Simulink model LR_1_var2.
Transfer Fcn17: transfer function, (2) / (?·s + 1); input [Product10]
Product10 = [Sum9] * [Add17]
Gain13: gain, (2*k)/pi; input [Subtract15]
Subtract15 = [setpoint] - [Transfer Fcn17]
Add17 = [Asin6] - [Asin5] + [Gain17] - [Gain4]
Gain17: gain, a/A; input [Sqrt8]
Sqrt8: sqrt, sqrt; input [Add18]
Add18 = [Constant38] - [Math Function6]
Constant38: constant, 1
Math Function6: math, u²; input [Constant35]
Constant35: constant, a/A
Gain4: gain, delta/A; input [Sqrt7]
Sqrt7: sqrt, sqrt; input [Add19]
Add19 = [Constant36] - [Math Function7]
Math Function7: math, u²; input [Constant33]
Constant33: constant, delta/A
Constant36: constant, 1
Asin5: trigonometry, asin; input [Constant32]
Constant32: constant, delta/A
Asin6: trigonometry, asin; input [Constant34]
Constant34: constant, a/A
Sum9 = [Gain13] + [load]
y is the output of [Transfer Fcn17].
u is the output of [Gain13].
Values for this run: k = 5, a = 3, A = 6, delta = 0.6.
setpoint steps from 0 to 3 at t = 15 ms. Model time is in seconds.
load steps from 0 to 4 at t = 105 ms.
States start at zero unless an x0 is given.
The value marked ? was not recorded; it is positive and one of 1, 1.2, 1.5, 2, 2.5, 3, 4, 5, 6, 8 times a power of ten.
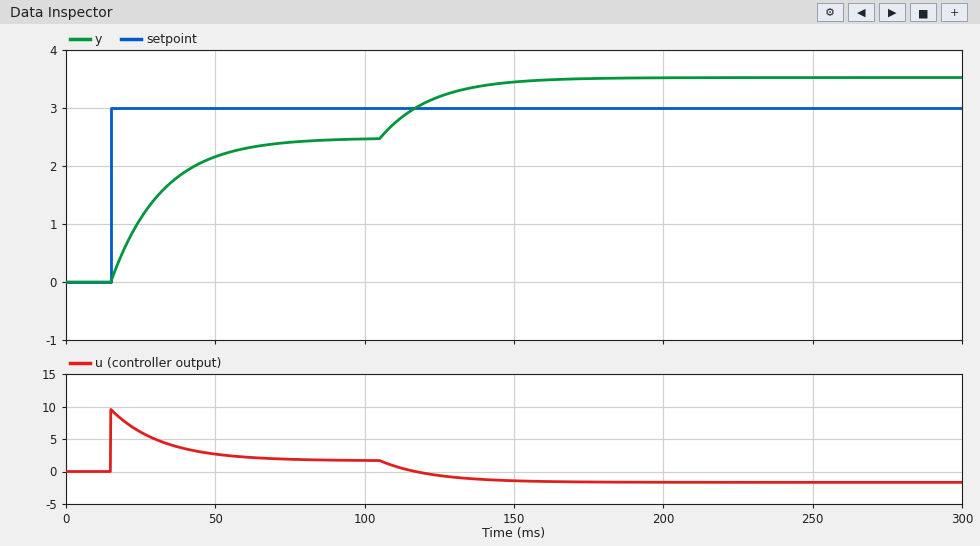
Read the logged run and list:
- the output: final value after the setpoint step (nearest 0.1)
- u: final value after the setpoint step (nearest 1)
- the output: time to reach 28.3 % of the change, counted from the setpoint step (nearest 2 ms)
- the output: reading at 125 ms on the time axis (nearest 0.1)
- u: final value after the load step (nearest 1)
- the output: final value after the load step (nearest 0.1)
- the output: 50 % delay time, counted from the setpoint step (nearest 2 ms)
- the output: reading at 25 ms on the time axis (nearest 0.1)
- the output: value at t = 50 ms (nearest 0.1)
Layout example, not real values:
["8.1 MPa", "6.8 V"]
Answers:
["2.5", "2", "6 ms", "3.2", "-2", "3.5", "12 ms", "1.1", "2.2"]
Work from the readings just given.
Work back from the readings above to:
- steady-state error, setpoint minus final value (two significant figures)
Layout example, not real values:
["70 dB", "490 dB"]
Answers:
["0.50"]
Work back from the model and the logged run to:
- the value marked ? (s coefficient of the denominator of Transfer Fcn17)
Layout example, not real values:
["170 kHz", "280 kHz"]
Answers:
["0.1"]
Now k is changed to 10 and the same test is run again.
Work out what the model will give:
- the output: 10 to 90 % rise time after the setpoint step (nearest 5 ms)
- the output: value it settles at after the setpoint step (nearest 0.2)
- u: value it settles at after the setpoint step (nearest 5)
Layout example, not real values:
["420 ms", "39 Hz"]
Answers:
["20 ms", "2.8", "0"]
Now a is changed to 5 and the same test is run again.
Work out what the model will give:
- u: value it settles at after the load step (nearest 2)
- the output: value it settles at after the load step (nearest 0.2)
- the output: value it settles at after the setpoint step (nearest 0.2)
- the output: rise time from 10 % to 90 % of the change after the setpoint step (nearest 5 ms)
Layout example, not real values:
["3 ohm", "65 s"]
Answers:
["-2", "3.8", "2.6", "25 ms"]
